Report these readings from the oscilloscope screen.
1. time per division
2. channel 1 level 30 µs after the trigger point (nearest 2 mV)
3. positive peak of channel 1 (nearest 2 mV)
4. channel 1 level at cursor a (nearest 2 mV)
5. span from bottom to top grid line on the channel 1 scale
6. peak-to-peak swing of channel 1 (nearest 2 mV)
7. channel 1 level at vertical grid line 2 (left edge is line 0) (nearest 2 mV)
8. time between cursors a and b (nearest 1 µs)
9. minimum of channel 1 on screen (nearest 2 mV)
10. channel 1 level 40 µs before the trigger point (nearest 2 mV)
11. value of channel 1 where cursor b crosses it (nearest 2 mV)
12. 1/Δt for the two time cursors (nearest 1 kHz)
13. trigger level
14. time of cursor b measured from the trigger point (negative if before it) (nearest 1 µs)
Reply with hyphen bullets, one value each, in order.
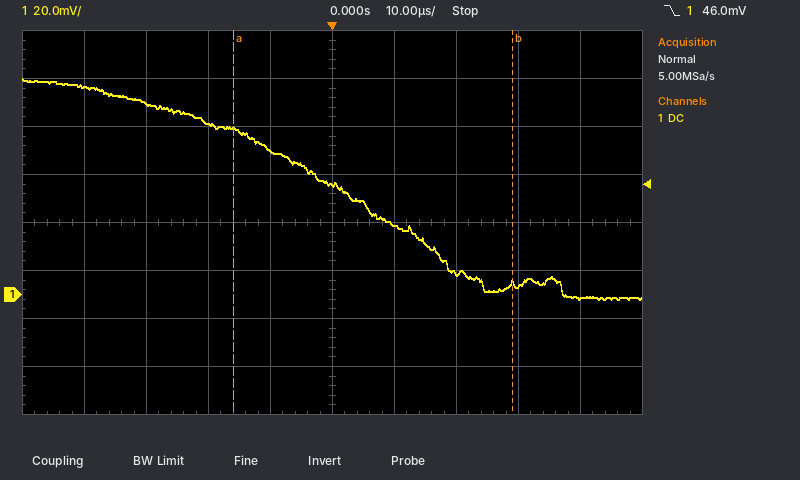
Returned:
- 10 µs
- 4 mV
- 90 mV
- 70 mV
- 160 mV
- 92 mV
- 80 mV
- 45 µs
- -2 mV
- 86 mV
- 4 mV
- 22 kHz
- 46.0 mV
- +29 µs
